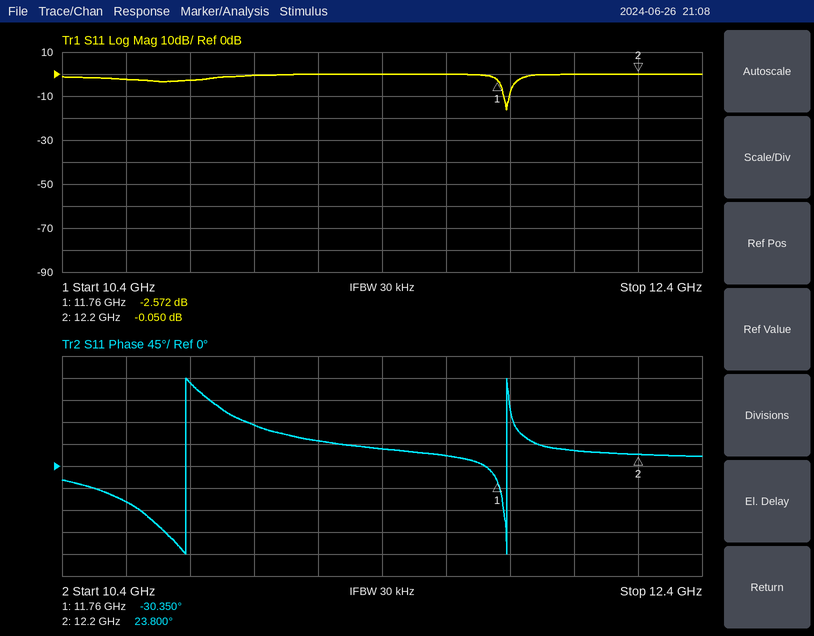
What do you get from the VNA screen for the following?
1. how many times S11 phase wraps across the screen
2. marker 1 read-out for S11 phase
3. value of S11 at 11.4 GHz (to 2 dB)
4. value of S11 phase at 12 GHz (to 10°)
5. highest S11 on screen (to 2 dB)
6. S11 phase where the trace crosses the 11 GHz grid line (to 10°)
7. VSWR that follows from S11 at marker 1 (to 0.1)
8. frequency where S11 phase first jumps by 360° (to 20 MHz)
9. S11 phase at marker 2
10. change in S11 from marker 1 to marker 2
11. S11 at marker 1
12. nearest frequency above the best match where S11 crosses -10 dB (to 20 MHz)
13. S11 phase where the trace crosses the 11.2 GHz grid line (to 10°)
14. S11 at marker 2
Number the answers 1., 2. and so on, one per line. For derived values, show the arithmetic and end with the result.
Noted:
1. 2
2. -30.350°
3. 0 dB
4. 30°
5. 0 dB
6. 80°
7. (1 + 0.7437)/(1 − 0.7437) ≈ 6.8
8. 10.78 GHz
9. 23.800°
10. -0.05 − (-2.572) = 2.522 dB
11. -2.572 dB
12. 11.80 GHz
13. 50°
14. -0.050 dB
